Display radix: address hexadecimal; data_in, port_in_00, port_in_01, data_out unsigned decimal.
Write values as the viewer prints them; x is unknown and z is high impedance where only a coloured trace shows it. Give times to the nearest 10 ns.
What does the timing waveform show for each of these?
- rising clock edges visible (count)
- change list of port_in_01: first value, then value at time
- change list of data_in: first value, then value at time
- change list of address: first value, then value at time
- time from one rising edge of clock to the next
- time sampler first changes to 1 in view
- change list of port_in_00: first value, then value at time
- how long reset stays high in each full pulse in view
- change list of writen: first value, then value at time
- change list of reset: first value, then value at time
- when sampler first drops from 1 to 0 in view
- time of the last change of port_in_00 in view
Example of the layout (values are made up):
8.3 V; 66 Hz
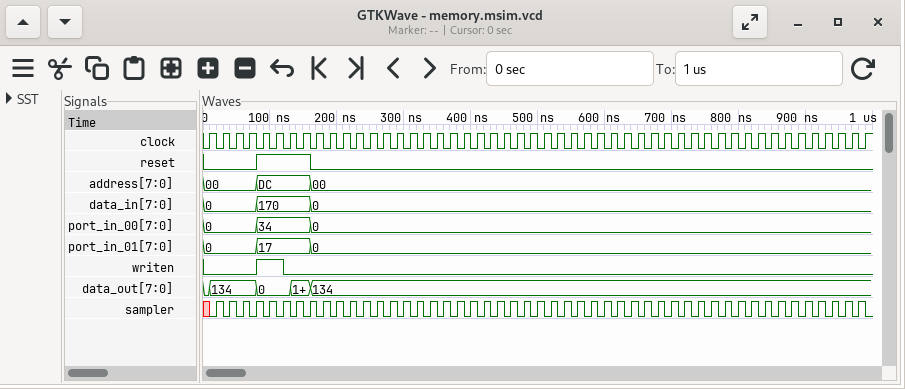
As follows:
50; 0, 17 at 80 ns, 0 at 160 ns; 0, 170 at 80 ns, 0 at 160 ns; 00, DC at 80 ns, 00 at 160 ns; 20 ns; 20 ns; 0, 34 at 80 ns, 0 at 160 ns; 80 ns; 0, 1 at 80 ns, 0 at 120 ns; 0, 1 at 80 ns, 0 at 160 ns; 30 ns; 160 ns
